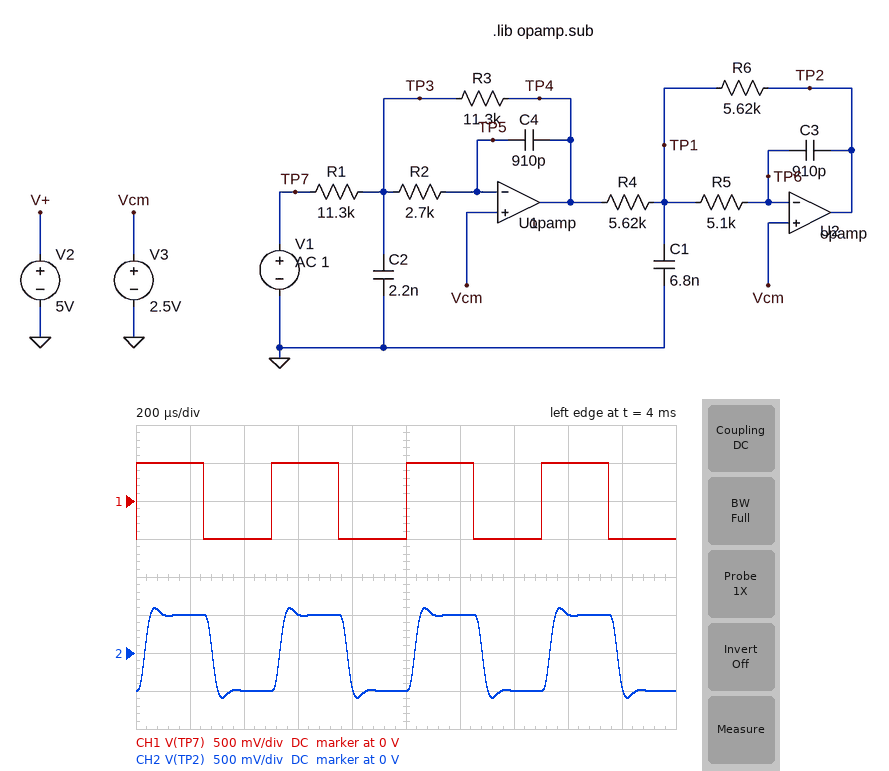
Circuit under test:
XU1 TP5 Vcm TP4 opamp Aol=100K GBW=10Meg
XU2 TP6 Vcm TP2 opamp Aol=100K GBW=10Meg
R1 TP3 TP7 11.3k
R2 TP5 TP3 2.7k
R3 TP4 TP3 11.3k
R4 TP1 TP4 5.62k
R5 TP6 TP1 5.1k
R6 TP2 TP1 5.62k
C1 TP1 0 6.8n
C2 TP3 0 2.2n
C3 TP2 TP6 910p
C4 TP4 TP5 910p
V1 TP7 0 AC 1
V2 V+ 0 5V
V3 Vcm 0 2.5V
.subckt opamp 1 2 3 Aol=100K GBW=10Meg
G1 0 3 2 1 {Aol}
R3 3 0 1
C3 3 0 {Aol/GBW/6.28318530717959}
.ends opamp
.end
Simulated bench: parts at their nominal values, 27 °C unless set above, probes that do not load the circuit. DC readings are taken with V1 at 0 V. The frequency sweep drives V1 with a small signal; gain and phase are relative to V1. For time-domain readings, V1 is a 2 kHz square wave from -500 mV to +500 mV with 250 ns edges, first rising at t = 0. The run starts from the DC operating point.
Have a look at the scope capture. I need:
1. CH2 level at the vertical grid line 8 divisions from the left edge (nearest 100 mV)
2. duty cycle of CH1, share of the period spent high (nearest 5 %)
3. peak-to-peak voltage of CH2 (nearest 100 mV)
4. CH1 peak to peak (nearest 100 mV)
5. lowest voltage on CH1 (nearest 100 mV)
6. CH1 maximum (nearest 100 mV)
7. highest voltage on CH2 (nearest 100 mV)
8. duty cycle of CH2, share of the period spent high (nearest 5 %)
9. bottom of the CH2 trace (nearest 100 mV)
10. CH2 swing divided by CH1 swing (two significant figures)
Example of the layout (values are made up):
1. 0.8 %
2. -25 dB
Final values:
1. 500 mV
2. 50 %
3. 1.2 V
4. 1.0 V
5. -500 mV
6. 500 mV
7. 600 mV
8. 50 %
9. -600 mV
10. 1.2
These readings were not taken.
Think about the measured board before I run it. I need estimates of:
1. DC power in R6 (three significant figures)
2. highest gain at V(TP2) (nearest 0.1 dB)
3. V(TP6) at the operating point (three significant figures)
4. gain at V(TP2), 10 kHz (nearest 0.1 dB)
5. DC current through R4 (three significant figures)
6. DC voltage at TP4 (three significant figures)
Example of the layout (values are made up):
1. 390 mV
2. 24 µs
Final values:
1. 1.11 mW
2. 0.1 dB
3. 2.50 V
4. -1.3 dB
5. 445 µA
6. 5.00 V
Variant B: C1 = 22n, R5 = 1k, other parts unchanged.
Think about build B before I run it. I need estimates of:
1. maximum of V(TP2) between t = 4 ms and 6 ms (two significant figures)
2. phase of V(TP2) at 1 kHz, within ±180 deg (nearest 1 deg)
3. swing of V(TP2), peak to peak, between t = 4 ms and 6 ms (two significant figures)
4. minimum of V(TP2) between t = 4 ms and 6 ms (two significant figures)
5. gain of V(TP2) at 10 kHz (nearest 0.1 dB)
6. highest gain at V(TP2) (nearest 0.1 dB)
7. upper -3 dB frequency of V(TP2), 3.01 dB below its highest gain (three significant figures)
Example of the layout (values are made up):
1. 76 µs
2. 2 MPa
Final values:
1. 700 mV
2. -8 deg
3. 1.4 V
4. -700 mV
5. 1.4 dB
6. 1.6 dB
7. 16.3 kHz
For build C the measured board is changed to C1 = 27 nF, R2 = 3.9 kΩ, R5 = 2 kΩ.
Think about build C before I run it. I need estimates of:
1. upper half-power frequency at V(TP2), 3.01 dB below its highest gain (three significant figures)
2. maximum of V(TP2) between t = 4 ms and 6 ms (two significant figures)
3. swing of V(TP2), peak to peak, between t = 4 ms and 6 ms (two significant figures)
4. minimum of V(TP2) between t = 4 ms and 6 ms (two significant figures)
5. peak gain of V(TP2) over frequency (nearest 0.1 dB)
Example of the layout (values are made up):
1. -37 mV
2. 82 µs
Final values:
1. 10.8 kHz
2. 830 mV
3. 1.7 V
4. -830 mV
5. 4.3 dB
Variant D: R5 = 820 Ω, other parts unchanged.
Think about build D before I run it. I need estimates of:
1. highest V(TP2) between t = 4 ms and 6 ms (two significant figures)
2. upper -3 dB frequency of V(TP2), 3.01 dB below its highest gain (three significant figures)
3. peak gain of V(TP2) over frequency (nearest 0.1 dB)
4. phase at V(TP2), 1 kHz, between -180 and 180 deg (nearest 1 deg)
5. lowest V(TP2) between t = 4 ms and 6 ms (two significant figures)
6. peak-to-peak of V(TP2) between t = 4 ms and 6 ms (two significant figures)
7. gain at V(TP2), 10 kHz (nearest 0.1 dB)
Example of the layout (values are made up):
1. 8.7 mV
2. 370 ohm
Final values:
1. 500 mV
2. 14.3 kHz
3. 0 dB
4. -8 deg
5. -500 mV
6. 1.0 V
7. -1.5 dB
